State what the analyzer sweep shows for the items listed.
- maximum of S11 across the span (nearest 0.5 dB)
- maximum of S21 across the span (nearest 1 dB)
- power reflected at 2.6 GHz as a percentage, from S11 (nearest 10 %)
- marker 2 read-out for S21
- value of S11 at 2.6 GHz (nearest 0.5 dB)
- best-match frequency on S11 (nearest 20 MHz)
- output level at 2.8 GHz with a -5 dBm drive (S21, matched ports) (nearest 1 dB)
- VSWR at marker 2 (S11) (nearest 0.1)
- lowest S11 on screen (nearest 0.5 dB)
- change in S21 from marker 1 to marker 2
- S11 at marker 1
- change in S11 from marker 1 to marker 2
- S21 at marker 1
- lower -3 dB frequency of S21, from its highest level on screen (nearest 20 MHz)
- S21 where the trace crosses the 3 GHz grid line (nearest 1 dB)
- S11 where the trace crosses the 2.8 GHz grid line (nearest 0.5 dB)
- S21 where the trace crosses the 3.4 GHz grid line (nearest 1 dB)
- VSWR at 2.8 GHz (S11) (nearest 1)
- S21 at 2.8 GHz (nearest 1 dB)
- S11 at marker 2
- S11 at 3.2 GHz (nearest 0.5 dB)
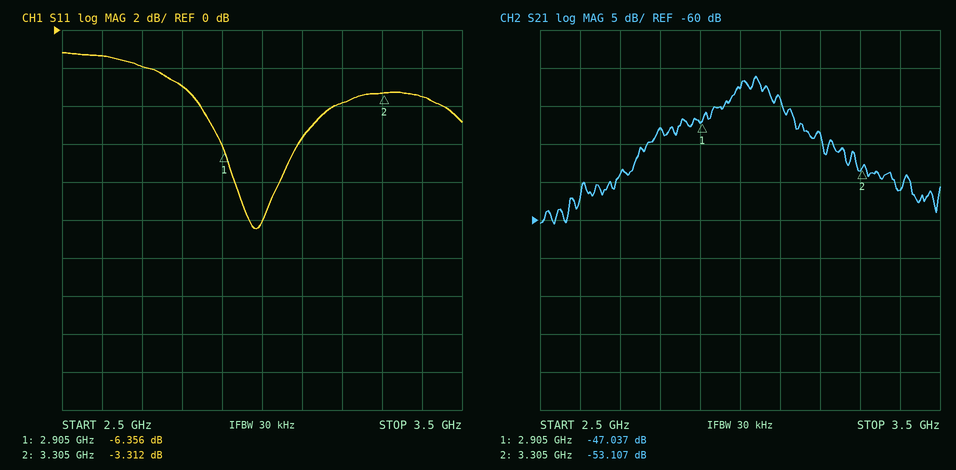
-1.0 dB
-41 dB
70 %
-53.107 dB
-1.5 dB
2.98 GHz
-53 dBm
5.3
-10.5 dB
-6.070 dB
-6.356 dB
3.044 dB
-47.037 dB
2.98 GHz
-43 dB
-3.0 dB
-56 dB
6
-48 dB
-3.312 dB
-4.0 dB
